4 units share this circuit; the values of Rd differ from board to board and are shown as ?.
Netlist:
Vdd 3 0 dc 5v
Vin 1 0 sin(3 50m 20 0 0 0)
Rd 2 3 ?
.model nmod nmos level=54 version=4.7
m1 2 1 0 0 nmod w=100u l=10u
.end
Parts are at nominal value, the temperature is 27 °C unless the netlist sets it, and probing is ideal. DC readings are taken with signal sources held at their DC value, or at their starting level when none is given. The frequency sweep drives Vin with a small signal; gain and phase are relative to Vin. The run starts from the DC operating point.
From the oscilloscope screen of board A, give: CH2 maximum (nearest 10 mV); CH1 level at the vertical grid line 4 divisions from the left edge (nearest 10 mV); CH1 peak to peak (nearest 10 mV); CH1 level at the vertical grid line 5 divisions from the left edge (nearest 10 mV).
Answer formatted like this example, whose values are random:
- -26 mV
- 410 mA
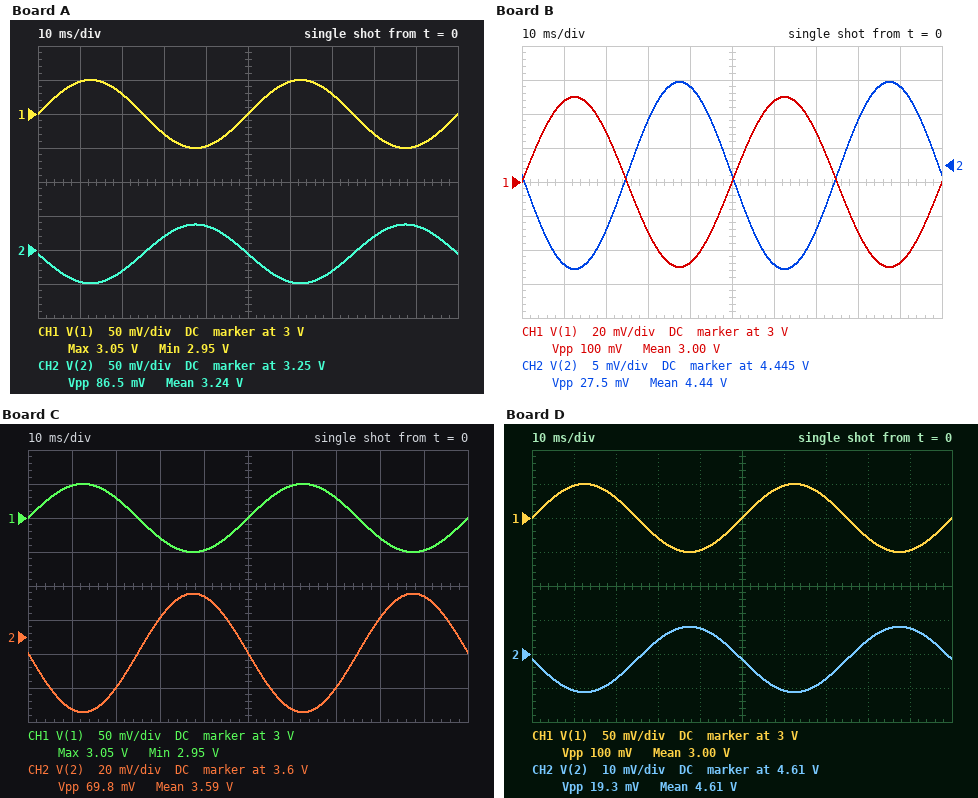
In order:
- 3.29 V
- 2.95 V
- 100 mV
- 3.00 V
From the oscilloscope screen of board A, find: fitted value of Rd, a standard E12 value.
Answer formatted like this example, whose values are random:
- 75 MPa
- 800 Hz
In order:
- 150 Ω
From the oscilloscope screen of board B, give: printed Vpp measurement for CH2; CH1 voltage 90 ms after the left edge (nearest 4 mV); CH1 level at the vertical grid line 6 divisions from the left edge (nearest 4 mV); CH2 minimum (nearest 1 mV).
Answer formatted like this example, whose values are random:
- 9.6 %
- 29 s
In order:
- 27.5 mV
- 2.952 V
- 3.048 V
- 4.430 V
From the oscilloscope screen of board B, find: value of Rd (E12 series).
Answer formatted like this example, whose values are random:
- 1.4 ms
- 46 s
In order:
- 47 Ω
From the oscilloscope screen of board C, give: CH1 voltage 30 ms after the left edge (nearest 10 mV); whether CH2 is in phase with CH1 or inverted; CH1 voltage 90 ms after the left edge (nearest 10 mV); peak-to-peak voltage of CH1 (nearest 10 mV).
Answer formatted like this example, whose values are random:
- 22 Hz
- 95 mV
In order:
- 2.97 V
- inverted
- 2.95 V
- 100 mV
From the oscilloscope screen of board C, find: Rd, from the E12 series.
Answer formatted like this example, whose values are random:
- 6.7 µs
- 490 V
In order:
- 120 Ω
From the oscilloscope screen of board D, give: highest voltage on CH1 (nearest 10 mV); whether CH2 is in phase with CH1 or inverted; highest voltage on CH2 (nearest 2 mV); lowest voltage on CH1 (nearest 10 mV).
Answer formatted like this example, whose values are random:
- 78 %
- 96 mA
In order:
- 3.05 V
- inverted
- 4.618 V
- 2.95 V
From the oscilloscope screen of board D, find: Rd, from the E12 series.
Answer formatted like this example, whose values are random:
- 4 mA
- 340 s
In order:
- 33 Ω
